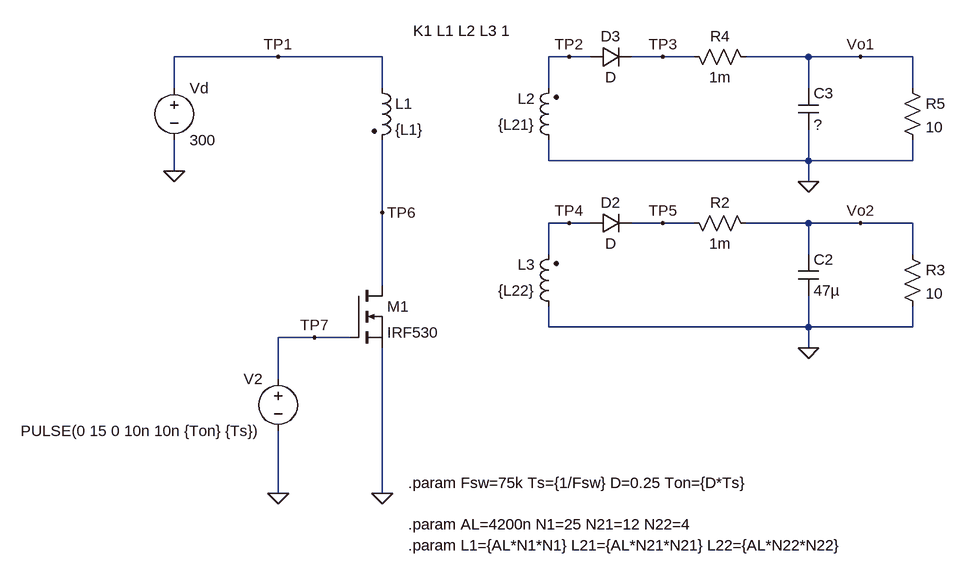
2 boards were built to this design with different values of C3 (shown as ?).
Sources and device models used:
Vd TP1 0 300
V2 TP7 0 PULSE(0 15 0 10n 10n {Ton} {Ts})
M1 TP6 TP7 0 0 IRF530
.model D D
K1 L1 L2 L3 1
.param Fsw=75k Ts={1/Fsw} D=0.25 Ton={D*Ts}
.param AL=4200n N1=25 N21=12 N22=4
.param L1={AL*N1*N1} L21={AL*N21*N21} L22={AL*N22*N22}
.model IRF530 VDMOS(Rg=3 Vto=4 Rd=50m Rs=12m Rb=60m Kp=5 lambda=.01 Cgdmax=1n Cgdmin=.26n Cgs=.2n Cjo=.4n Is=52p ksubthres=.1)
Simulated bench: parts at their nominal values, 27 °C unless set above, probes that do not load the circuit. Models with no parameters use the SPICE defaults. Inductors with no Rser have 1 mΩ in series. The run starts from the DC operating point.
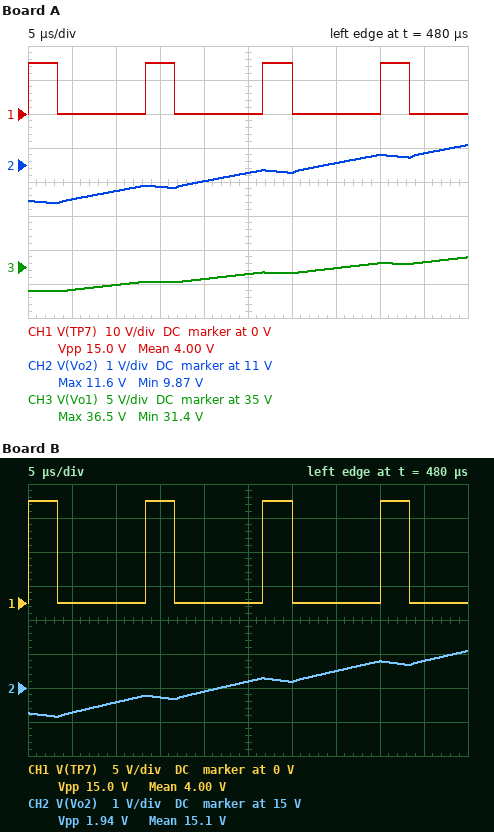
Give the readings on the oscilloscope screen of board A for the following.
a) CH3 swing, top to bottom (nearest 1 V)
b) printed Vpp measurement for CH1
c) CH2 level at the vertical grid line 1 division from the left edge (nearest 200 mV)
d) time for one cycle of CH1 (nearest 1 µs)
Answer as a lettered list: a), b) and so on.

a) 5 V
b) 15.0 V
c) 10.0 V
d) 13 µs
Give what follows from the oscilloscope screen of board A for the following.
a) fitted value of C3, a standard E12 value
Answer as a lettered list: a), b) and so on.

a) 120 µF
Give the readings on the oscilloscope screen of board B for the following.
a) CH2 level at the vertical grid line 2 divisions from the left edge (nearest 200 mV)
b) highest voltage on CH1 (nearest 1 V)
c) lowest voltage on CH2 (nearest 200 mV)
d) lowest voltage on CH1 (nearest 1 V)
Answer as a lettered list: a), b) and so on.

a) 14.6 V
b) 15 V
c) 14.2 V
d) 0 V
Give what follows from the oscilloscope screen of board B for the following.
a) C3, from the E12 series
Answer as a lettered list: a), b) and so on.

a) 68 µF
